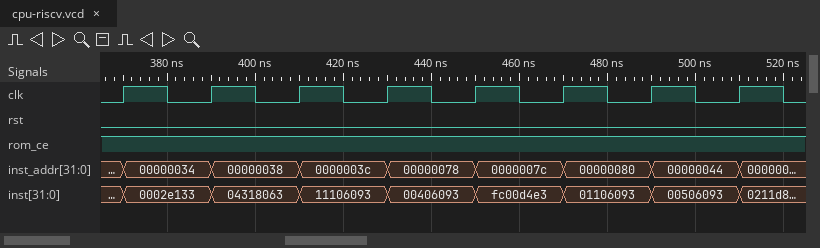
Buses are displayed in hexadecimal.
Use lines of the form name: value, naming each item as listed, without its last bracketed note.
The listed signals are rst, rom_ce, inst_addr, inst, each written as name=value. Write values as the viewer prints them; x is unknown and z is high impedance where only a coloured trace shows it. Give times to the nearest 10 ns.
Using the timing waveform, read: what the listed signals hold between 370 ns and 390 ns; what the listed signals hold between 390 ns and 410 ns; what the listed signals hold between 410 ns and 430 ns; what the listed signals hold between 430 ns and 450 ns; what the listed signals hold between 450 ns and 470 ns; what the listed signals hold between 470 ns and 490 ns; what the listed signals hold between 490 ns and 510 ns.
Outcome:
what the listed signals hold between 370 ns and 390 ns: rst=0, rom_ce=1, inst_addr=00000034, inst=0002e133
what the listed signals hold between 390 ns and 410 ns: rst=0, rom_ce=1, inst_addr=00000038, inst=04318063
what the listed signals hold between 410 ns and 430 ns: rst=0, rom_ce=1, inst_addr=0000003c, inst=11106093
what the listed signals hold between 430 ns and 450 ns: rst=0, rom_ce=1, inst_addr=00000078, inst=00406093
what the listed signals hold between 450 ns and 470 ns: rst=0, rom_ce=1, inst_addr=0000007c, inst=fc00d4e3
what the listed signals hold between 470 ns and 490 ns: rst=0, rom_ce=1, inst_addr=00000080, inst=01106093
what the listed signals hold between 490 ns and 510 ns: rst=0, rom_ce=1, inst_addr=00000044, inst=00506093
